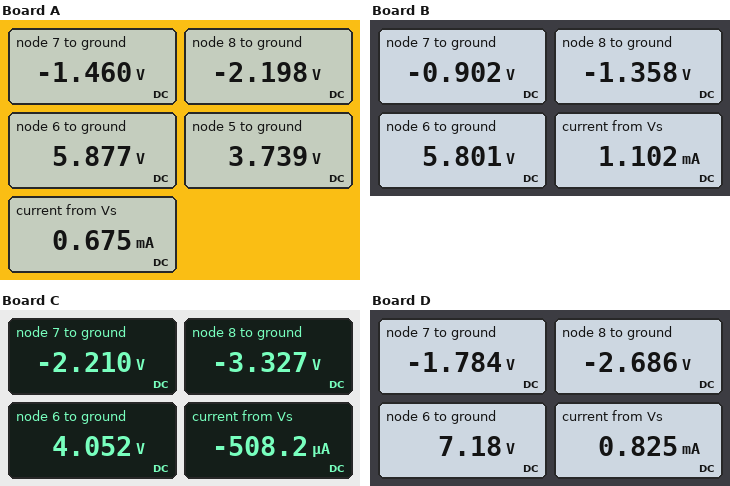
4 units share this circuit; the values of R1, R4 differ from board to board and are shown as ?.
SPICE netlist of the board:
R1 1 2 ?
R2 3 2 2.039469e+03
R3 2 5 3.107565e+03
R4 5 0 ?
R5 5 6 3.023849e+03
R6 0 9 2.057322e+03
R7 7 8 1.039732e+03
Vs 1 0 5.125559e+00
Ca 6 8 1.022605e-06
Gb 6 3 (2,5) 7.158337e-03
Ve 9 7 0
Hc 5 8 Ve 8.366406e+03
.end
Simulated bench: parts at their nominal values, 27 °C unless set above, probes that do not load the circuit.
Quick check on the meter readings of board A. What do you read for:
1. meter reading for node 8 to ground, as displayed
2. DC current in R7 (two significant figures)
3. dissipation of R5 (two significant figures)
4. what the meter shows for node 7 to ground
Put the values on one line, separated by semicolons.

-2.198 V; 710 µA; 1.5 mW; -1.460 V
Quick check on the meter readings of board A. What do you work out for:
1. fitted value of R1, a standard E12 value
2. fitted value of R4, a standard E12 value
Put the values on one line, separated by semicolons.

2.2 kΩ; 2.7 kΩ
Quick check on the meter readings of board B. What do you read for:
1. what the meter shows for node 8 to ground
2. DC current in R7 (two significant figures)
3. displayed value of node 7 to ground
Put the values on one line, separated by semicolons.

-1.358 V; 440 µA; -0.902 V
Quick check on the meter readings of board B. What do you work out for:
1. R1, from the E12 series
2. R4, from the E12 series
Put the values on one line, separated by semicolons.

2.7 kΩ; 1.5 kΩ
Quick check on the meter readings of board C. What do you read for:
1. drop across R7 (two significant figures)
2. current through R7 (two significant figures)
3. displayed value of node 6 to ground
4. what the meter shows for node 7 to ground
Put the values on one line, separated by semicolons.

1.1 V; 1.1 mA; 4.052 V; -2.210 V
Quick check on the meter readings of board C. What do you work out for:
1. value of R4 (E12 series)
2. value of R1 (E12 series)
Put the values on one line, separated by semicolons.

10 kΩ; 1.2 kΩ
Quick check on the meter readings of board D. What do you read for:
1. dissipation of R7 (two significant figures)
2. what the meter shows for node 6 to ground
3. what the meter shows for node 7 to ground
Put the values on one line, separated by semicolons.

780 µW; 7.18 V; -1.784 V
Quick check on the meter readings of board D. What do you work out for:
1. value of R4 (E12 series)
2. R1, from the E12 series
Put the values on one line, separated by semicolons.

2.7 kΩ; 820 Ω
